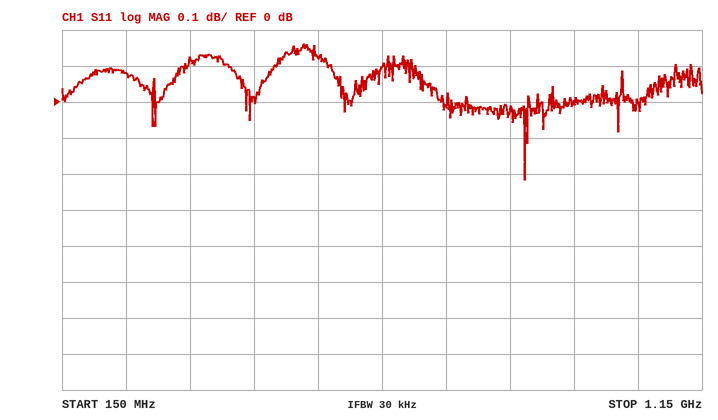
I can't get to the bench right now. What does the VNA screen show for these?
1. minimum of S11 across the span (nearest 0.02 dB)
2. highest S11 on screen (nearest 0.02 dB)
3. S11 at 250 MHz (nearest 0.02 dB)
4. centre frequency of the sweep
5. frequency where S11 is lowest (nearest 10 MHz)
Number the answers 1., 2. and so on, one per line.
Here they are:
1. -0.22 dB
2. 0.16 dB
3. 0.08 dB
4. 650 MHz
5. 870 MHz
